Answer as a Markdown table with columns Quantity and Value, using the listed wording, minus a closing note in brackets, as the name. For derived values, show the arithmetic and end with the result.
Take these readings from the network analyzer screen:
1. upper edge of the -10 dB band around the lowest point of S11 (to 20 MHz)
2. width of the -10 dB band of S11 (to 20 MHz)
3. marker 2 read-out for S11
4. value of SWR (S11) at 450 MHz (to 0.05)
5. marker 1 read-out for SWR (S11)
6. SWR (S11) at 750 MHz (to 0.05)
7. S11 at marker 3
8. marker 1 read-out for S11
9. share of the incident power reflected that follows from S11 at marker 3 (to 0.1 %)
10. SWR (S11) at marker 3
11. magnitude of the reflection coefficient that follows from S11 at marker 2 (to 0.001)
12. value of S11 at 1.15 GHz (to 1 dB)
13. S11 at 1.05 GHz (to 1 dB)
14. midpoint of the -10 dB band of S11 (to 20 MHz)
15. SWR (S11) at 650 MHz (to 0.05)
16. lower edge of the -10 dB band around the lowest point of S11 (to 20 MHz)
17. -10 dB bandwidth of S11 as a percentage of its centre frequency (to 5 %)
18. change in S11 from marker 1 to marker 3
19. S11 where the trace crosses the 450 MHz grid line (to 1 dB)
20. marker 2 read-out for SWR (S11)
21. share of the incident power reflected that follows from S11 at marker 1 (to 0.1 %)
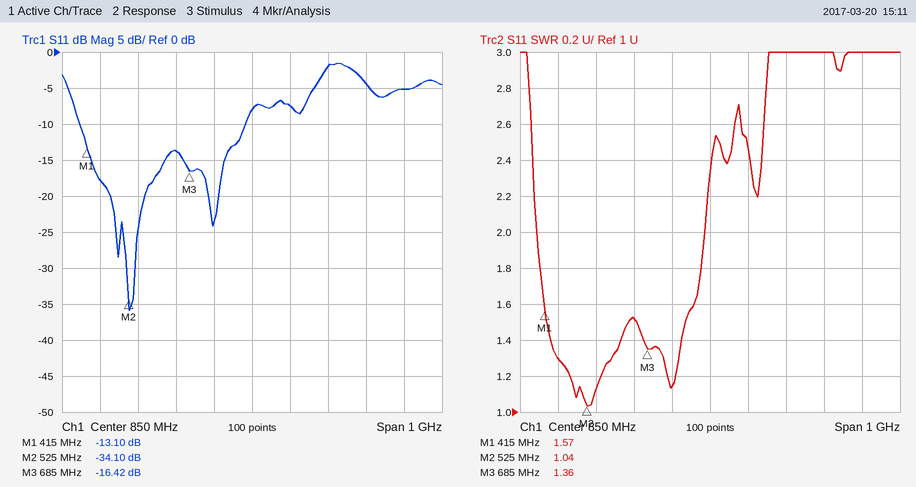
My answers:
| Quantity | Value |
|---|---|
| upper edge of the -10 dB band around the lowest point of S11 | 840 MHz |
| width of the -10 dB band of S11 | 840 MHz − 400 MHz = 440 MHz |
| marker 2 read-out for S11 | -34.10 dB |
| value of SWR (S11) at 450 MHz | 1.30 |
| marker 1 read-out for SWR | 1.57 |
| SWR (S11) at 750 MHz | 1.15 |
| S11 at marker 3 | -16.42 dB |
| marker 1 read-out for S11 | -13.10 dB |
| share of the incident power reflected that follows from S11 at marker 3 | 10^(-16.42/10) ≈ 2.3 % |
| SWR (S11) at marker 3 | 1.36 |
| magnitude of the reflection coefficient that follows from S11 at marker 2 | 10^(-34.1/20) ≈ 0.020 |
| value of S11 at 1.15 GHz | -4 dB |
| S11 at 1.05 GHz | -2 dB |
| midpoint of the -10 dB band of S11 | 620 MHz |
| SWR (S11) at 650 MHz | 1.50 |
| lower edge of the -10 dB band around the lowest point of S11 | 400 MHz |
| -10 dB bandwidth of S11 as a percentage of its centre frequency | 440 MHz / 620 MHz ≈ 71.0 %, so 70 % to the nearest 5 % |
| change in S11 from marker 1 to marker 3 | -16.42 − (-13.1) = -3.32 dB |
| S11 where the trace crosses the 450 MHz grid line | -18 dB |
| marker 2 read-out for SWR | 1.04 |
| share of the incident power reflected that follows from S11 at marker 1 | 10^(-13.1/10) ≈ 4.9 % |
